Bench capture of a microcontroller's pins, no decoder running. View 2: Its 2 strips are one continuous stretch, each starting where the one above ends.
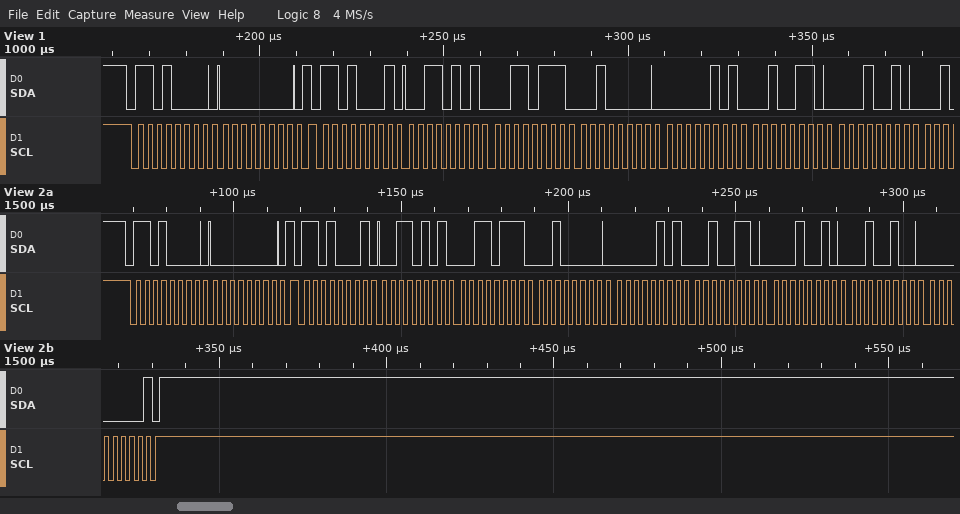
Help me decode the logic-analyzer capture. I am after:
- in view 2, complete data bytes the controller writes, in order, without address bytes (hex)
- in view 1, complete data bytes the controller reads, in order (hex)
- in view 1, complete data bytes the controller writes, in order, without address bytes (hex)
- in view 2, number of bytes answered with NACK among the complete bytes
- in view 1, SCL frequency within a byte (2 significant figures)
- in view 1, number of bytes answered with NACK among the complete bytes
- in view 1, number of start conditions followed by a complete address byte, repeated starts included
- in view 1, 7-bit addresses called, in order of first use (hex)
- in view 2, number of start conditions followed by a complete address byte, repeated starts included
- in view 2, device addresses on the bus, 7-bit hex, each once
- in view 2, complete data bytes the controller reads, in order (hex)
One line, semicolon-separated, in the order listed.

00; 35 37 20 05 26 12; 00; 1; 400 kHz; 0; 2; 0x68; 2; 0x68; 35 37 20 05 26 12 24 00
